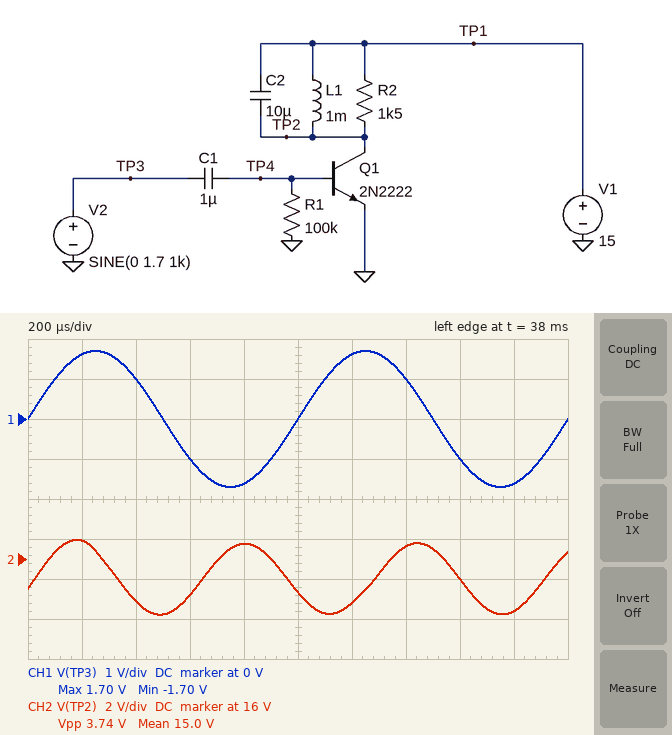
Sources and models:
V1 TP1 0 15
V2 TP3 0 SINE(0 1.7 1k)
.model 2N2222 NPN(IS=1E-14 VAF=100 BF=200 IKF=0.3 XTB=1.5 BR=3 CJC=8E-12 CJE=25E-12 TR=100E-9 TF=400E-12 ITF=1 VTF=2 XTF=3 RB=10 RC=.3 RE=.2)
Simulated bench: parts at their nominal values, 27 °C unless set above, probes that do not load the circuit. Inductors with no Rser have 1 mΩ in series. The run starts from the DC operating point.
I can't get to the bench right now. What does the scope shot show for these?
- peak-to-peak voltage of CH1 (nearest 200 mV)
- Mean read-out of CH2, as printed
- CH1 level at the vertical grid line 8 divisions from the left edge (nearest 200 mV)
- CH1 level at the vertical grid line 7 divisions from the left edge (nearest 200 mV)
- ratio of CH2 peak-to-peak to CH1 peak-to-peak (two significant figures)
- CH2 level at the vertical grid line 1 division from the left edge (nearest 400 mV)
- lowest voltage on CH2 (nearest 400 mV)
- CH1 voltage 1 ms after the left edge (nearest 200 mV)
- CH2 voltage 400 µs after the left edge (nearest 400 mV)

3.4 V
15.0 V
-1.0 V
1.0 V
1.1
16.8 V
13.2 V
0 V
14.0 V
